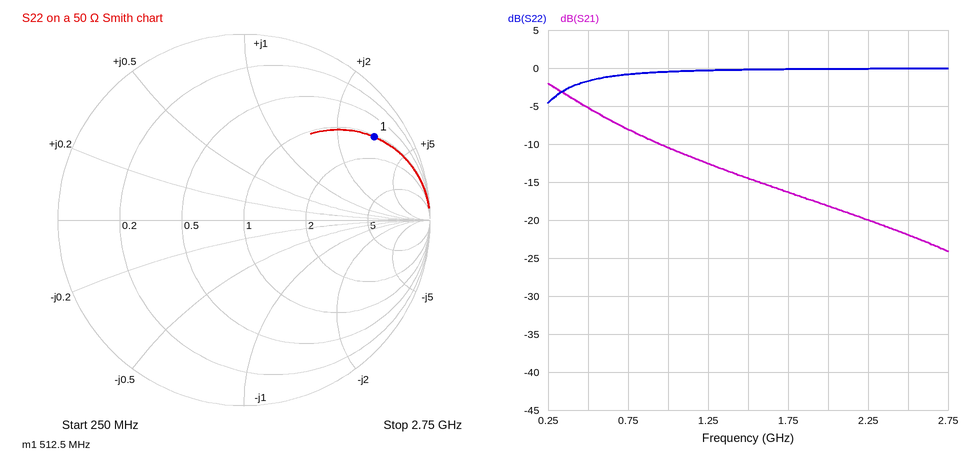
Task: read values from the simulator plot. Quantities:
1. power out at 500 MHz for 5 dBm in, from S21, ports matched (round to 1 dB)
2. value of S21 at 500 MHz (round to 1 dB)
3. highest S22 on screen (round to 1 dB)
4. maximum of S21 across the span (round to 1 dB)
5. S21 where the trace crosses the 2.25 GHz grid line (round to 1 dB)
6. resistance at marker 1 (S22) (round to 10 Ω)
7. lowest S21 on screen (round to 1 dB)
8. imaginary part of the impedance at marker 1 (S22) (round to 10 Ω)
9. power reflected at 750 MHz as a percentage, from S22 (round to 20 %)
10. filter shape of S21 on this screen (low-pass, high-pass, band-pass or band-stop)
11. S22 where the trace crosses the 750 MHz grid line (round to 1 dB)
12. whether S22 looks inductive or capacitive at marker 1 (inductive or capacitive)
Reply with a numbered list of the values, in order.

1. 0 dBm
2. -5 dB
3. 0 dB
4. -2 dB
5. -20 dB
6. 50 Ω
7. -24 dB
8. +150 Ω
9. 80 %
10. low-pass
11. -1 dB
12. inductive
